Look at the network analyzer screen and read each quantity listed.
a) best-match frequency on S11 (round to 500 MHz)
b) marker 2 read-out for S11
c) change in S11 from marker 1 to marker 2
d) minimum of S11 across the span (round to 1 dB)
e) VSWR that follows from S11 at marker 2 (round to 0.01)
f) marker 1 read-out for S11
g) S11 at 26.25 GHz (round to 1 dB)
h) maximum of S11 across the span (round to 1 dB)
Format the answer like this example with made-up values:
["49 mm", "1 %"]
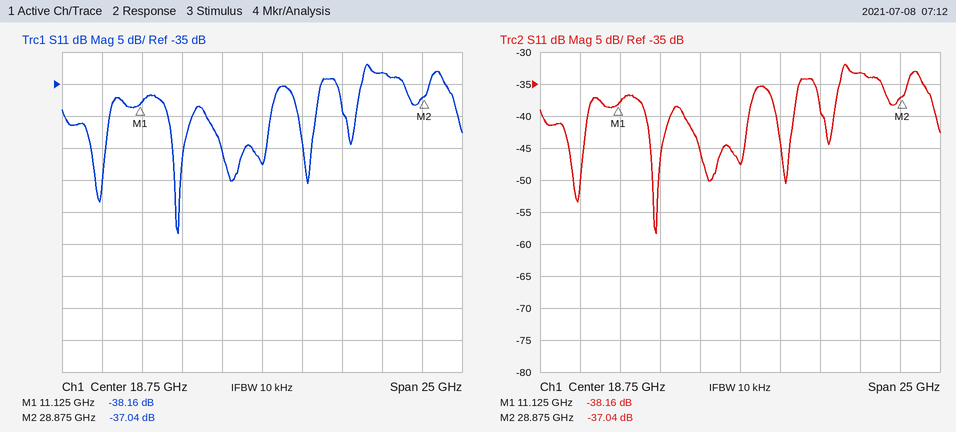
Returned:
["13.5 GHz", "-37.04 dB", "1.12 dB", "-58 dB", "1.03", "-38.16 dB", "-33 dB", "-32 dB"]
